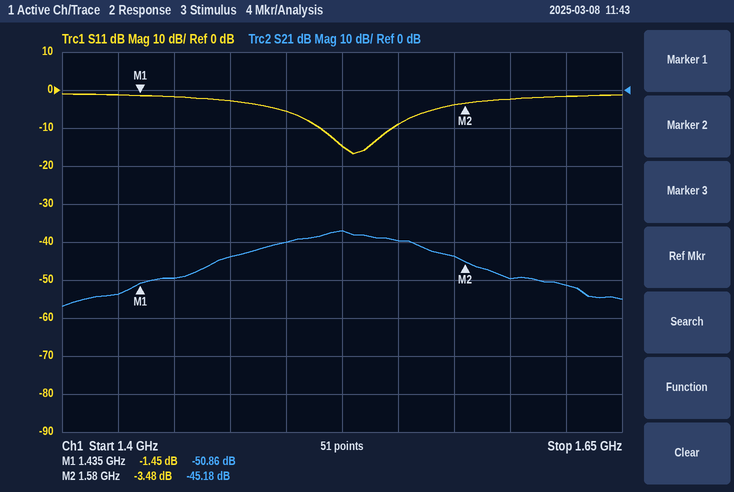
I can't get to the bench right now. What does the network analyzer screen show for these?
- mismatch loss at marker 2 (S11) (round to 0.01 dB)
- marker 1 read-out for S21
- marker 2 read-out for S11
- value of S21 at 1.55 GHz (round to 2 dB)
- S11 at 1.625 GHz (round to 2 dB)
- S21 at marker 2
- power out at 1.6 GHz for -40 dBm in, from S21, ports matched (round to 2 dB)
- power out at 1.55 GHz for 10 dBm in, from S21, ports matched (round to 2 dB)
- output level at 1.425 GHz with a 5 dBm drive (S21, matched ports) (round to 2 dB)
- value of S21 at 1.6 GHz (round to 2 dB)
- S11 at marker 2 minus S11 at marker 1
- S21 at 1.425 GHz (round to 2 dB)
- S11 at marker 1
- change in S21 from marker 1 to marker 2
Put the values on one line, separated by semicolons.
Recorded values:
2.59 dB; -50.86 dB; -3.48 dB; -40 dB; -2 dB; -45.18 dB; -90 dBm; -30 dBm; -48 dBm; -50 dB; -2.03 dB; -54 dB; -1.45 dB; 5.68 dB
